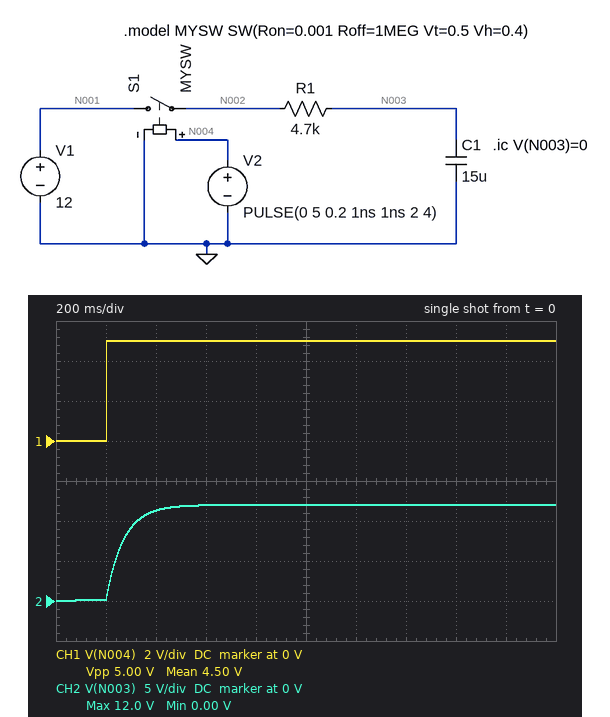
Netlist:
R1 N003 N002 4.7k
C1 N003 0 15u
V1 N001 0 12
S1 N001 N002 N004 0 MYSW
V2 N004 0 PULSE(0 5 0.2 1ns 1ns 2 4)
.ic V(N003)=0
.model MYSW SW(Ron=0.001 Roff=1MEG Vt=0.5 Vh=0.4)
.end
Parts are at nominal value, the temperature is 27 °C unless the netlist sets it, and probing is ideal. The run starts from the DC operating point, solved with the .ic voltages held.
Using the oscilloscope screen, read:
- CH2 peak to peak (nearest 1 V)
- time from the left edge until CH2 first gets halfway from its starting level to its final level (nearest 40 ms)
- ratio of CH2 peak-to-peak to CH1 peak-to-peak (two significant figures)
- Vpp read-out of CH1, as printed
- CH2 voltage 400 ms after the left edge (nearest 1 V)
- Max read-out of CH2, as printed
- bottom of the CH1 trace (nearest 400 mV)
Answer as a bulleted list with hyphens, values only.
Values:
- 12 V
- 240 ms
- 2.4
- 5.00 V
- 11 V
- 12.0 V
- 0 V
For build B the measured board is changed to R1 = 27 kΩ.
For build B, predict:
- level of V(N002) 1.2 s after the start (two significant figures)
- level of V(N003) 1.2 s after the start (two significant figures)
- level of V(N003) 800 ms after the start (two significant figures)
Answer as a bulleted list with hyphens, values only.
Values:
- 12 V
- 11 V
- 9.3 V
